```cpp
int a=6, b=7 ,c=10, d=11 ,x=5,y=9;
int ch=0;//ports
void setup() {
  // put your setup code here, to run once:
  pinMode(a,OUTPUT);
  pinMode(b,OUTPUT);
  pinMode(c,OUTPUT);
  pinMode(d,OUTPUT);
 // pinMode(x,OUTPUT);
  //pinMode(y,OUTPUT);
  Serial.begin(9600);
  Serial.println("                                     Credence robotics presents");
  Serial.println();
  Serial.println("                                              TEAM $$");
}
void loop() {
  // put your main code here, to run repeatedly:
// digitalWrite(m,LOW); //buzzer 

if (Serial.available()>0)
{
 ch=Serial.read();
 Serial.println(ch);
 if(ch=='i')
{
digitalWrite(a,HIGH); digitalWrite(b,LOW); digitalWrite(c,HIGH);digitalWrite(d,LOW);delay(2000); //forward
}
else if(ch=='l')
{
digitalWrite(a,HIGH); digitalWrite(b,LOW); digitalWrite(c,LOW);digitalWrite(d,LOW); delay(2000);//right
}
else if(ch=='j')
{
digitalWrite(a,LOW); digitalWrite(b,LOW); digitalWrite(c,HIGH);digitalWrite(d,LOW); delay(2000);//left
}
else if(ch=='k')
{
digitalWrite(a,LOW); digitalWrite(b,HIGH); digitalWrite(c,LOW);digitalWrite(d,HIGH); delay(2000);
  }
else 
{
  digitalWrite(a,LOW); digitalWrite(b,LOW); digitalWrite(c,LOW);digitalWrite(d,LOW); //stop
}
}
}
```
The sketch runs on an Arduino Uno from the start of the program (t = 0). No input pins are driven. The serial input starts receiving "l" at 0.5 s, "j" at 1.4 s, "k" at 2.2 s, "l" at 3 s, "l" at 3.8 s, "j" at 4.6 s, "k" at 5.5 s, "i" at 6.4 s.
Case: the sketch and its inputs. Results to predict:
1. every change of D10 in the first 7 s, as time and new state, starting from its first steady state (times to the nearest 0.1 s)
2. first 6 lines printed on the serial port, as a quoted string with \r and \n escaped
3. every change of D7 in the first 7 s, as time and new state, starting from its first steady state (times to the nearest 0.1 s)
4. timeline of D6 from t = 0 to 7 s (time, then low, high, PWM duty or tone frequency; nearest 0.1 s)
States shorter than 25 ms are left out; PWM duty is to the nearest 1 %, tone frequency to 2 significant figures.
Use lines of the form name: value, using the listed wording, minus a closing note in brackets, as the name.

every change of D10 in the first 7 s, as time and new state, starting from its first steady state: 0 s low; 2.5 s high; 4.5 s low
first 6 lines printed on the serial port, as a quoted string with \r and \n escaped: "                                     Credence robotics presents\r\n\r\n                                              TEAM $$\r\n108\r\n106\r\n107\r\n"
every change of D7 in the first 7 s, as time and new state, starting from its first steady state: 0 s low; 4.5 s high; 6.5 s low
timeline of D6 from t = 0 to 7 s: 0 s low; 0.5 s high; 2.5 s low; 6.5 s high
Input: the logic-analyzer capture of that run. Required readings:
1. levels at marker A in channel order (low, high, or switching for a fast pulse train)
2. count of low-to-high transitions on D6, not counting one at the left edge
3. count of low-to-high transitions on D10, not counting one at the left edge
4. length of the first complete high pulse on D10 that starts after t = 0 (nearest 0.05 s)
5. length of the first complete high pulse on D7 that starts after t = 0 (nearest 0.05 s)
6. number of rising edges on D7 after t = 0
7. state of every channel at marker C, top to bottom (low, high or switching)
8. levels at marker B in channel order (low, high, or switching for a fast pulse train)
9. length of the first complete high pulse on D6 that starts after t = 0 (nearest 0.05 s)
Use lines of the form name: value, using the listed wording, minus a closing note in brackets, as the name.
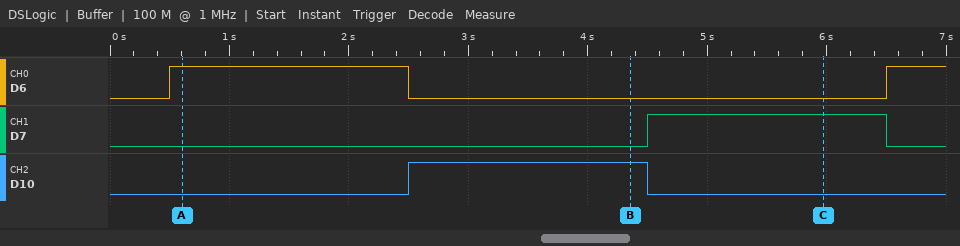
levels at marker A in channel order: D6 high, D7 low, D10 low
count of low-to-high transitions on D6, not counting one at the left edge: 2
count of low-to-high transitions on D10, not counting one at the left edge: 1
length of the first complete high pulse on D10 that starts after t = 0: 2.00 s
length of the first complete high pulse on D7 that starts after t = 0: 2.00 s
number of rising edges on D7 after t = 0: 1
state of every channel at marker C, top to bottom: D6 low, D7 high, D10 low
levels at marker B in channel order: D6 low, D7 low, D10 high
length of the first complete high pulse on D6 that starts after t = 0: 2.00 s
